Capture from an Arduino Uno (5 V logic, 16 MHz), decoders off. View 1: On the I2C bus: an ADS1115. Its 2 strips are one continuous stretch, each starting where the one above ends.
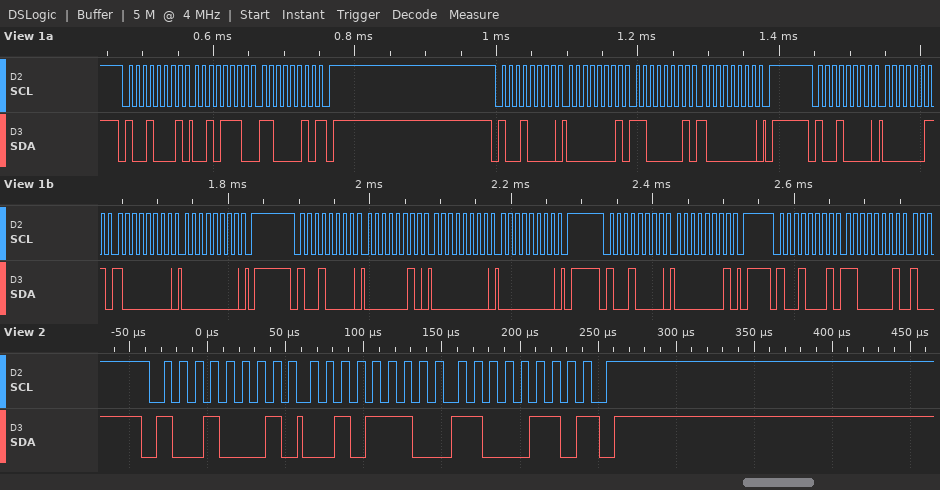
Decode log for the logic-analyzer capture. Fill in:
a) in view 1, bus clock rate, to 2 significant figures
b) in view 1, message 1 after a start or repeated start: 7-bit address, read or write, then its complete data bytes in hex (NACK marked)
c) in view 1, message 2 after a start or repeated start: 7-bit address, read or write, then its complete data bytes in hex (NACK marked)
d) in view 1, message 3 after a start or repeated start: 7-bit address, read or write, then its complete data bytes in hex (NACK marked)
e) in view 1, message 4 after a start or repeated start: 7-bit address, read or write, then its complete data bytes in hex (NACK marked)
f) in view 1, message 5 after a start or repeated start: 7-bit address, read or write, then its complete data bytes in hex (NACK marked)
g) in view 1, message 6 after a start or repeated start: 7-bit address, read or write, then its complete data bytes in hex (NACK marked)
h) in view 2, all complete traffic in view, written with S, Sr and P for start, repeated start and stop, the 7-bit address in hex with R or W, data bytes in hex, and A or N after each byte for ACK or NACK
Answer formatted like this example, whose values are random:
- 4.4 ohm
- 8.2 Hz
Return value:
- 100 kHz
- 0x48 read: 2E C2 NACK
- 0x48 write: 01 C1 80
- 0x48 write: 03 80 00
- 0x48 write: 02 00 00
- 0x48 write: 01
- 0x48 read: C1
- S 48R A 2E A C6 N P
